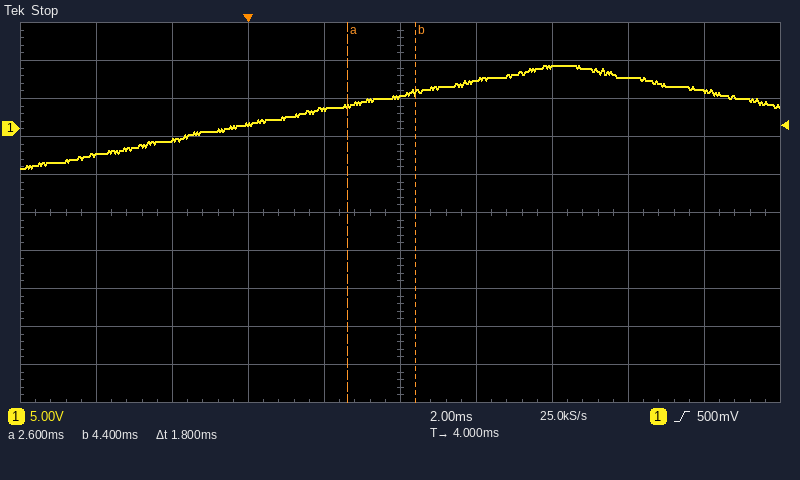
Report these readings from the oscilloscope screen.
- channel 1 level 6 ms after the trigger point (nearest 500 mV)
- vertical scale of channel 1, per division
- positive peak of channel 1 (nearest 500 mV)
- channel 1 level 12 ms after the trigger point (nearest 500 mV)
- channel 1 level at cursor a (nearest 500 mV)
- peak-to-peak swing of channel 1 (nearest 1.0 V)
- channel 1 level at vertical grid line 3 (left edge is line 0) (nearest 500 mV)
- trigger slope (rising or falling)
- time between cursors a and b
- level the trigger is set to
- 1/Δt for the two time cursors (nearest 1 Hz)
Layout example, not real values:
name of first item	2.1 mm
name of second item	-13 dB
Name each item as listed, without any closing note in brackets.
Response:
channel 1 level 6 ms after the trigger point	6.5 V
vertical scale of channel 1, per division	5 V
positive peak of channel 1	8.5 V
channel 1 level 12 ms after the trigger point	5.0 V
channel 1 level at cursor a	3.0 V
peak-to-peak swing of channel 1	14.0 V
channel 1 level at vertical grid line 3 (left edge is line 0)	500 mV
trigger slope	rising
time between cursors a and b	1.8 ms
level the trigger is set to	500 mV
1/Δt for the two time cursors	556 Hz
